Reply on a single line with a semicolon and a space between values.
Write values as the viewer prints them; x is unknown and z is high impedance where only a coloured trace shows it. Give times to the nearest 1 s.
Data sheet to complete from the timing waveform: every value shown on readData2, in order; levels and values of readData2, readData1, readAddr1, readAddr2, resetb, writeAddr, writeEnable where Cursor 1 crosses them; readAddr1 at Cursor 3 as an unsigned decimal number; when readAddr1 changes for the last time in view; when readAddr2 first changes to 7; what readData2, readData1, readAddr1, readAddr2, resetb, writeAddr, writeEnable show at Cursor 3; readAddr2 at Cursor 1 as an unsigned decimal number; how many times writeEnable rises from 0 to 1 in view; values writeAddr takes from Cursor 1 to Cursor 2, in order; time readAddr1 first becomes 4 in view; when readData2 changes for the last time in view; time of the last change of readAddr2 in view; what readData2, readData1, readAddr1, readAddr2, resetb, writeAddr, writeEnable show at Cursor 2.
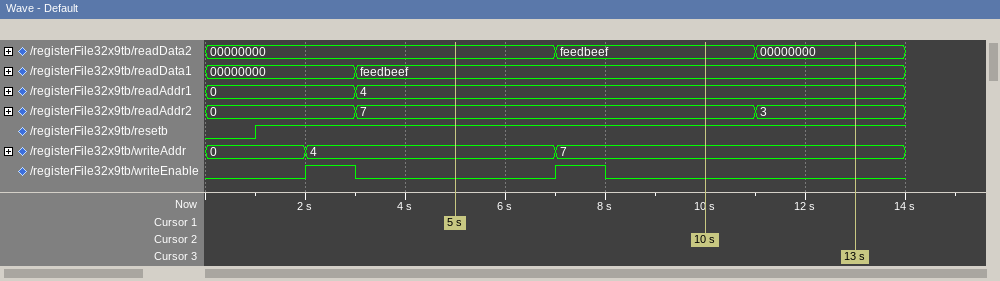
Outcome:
00000000, feedbeef, 00000000; readData2=00000000, readData1=feedbeef, readAddr1=4, readAddr2=7, resetb=1, writeAddr=4, writeEnable=0; 4; 3 s; 3 s; readData2=00000000, readData1=feedbeef, readAddr1=4, readAddr2=3, resetb=1, writeAddr=7, writeEnable=0; 7; 2; 4, 7; 3 s; 11 s; 11 s; readData2=feedbeef, readData1=feedbeef, readAddr1=4, readAddr2=7, resetb=1, writeAddr=7, writeEnable=0
